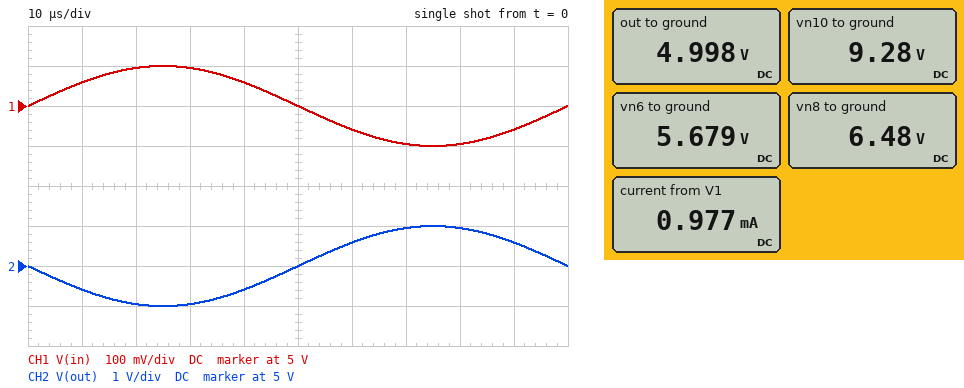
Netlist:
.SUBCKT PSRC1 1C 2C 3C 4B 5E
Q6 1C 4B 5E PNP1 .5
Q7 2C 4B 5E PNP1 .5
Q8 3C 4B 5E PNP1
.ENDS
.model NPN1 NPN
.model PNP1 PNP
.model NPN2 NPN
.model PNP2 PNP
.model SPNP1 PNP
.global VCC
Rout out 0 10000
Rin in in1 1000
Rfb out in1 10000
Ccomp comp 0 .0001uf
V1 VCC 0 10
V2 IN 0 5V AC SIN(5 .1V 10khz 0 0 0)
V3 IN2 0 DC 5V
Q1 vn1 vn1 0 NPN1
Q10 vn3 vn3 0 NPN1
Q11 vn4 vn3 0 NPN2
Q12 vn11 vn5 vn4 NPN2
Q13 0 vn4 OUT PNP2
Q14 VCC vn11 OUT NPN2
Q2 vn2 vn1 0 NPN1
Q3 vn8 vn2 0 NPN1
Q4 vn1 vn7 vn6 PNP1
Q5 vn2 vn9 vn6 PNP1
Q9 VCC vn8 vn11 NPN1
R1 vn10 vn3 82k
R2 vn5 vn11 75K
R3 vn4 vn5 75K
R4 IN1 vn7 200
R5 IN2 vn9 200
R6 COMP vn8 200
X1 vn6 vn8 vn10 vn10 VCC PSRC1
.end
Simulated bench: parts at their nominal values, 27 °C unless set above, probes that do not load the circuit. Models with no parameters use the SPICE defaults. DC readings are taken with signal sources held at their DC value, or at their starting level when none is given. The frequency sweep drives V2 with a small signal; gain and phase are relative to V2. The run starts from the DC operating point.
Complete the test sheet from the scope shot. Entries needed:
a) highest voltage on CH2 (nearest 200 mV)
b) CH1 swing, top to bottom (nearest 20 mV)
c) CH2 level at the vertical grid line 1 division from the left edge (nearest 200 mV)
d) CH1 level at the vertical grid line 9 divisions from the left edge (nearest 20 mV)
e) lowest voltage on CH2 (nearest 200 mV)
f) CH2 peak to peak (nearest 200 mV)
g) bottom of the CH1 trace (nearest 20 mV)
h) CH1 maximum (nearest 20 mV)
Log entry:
6.0 V
200 mV
4.4 V
4.94 V
4.0 V
2.0 V
4.90 V
5.10 V
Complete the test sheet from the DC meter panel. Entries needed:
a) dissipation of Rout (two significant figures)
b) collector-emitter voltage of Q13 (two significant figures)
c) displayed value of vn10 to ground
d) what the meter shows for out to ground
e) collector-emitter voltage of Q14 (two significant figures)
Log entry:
2.5 mW
-5.0 V
9.28 V
4.998 V
5.0 V
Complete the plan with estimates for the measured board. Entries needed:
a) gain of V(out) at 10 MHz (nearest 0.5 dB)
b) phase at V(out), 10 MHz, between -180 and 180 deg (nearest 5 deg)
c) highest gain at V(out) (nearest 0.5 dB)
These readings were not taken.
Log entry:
17.0 dB
170 deg
20.0 dB
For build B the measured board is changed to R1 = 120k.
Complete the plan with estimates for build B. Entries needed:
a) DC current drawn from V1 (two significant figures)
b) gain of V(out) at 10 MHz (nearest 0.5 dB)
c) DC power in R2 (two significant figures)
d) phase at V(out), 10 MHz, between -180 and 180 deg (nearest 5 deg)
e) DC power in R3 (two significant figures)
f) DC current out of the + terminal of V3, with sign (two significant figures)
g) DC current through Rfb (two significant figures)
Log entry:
750 µA
16.0 dB
7.4 µW
165 deg
6.6 µW
-170 nA
170 nA
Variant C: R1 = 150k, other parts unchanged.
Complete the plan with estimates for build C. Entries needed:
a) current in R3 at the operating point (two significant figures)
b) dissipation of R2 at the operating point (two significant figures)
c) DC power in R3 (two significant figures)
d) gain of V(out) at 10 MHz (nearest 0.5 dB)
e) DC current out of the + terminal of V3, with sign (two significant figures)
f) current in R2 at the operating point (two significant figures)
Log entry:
9.3 µA
7.1 µW
6.4 µW
15.5 dB
-140 nA
9.7 µA
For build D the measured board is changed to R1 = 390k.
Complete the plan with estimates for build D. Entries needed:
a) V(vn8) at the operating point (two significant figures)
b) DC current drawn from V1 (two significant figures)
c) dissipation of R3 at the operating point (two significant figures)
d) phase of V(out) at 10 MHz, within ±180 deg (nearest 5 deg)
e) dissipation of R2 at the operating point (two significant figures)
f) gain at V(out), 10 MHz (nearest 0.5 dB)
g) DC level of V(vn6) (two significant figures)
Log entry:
6.4 V
570 µA
5.8 µW
155 deg
6.0 µW
10.5 dB
5.6 V
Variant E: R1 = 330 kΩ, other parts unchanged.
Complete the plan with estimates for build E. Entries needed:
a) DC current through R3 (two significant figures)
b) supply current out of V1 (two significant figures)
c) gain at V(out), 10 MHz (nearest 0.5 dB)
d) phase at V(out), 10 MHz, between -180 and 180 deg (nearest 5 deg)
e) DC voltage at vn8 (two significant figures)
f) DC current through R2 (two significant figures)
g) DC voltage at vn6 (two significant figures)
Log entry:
8.9 µA
580 µA
11.5 dB
155 deg
6.4 V
9.1 µA
5.6 V
